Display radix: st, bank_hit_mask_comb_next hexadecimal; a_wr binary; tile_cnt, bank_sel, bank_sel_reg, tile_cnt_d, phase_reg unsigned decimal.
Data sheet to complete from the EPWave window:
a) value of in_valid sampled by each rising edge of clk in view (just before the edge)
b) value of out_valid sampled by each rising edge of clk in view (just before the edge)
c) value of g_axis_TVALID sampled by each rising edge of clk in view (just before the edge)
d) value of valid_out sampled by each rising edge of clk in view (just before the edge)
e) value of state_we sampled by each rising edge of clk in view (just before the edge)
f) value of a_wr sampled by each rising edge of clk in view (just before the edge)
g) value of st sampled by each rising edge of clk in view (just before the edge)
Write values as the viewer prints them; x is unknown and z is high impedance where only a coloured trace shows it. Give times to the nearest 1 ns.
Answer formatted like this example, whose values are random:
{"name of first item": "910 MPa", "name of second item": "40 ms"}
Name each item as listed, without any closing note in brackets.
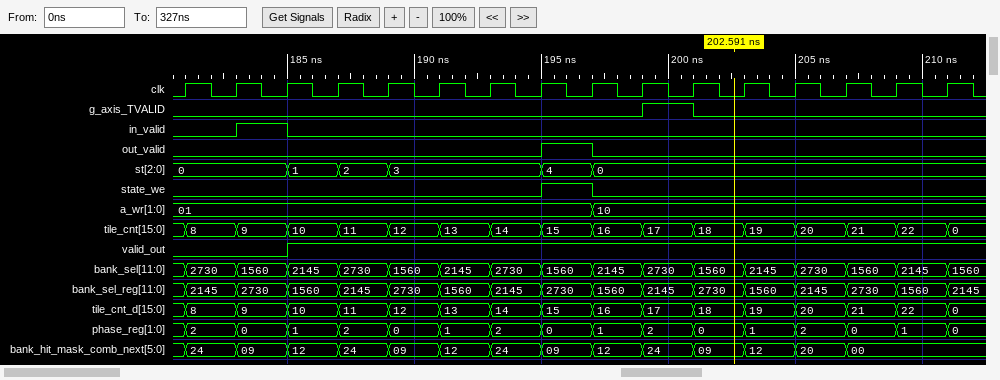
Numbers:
{"value of in_valid sampled by each rising edge of clk in view": "0 0 1 0 0 0 0 0 0 0 0 0 0 0 0 0", "value of out_valid sampled by each rising edge of clk in view": "0 0 0 0 0 0 0 0 1 0 0 0 0 0 0 0", "value of g_axis_TVALID sampled by each rising edge of clk in view": "0 0 0 0 0 0 0 0 0 0 1 0 0 0 0 0", "value of valid_out sampled by each rising edge of clk in view": "0 0 0 1 1 1 1 1 1 1 1 1 1 1 1 1", "value of state_we sampled by each rising edge of clk in view": "0 0 0 0 0 0 0 0 1 0 0 0 0 0 0 0", "value of a_wr sampled by each rising edge of clk in view": "01, 01, 01, 01, 01, 01, 01, 01, 01, 10, 10, 10, 10, 10, 10, 10", "value of st sampled by each rising edge of clk in view": "0, 0, 0, 1, 2, 3, 3, 3, 4, 0, 0, 0, 0, 0, 0, 0"}
